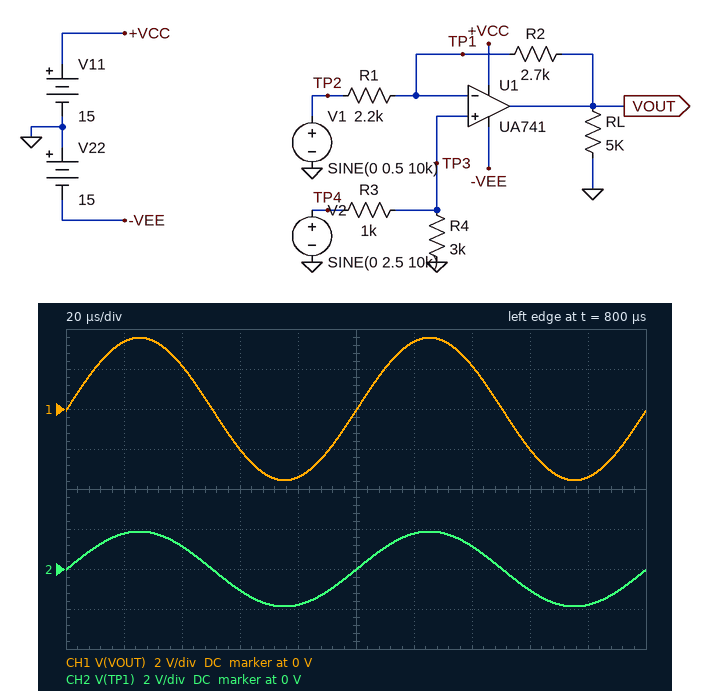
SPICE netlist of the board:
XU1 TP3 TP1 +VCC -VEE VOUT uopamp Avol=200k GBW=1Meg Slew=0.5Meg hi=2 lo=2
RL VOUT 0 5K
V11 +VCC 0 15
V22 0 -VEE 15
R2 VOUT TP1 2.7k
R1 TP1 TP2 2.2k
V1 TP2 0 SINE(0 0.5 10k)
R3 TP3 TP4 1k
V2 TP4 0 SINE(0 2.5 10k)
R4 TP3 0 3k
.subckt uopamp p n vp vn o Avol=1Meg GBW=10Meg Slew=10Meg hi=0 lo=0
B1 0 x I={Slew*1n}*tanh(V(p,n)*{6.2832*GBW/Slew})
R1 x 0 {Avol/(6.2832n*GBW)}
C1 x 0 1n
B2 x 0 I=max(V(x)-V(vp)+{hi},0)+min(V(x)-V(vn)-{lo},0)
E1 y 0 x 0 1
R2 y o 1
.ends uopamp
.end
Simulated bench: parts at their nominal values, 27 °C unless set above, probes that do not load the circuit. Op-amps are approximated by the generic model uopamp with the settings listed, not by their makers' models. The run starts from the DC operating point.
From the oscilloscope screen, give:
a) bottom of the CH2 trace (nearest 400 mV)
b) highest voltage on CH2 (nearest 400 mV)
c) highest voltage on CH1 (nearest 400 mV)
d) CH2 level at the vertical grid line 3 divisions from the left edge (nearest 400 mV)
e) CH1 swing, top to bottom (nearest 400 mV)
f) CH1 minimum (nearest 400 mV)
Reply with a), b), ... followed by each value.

a) -2.0 V
b) 2.0 V
c) 3.6 V
d) -1.2 V
e) 7.2 V
f) -3.6 V
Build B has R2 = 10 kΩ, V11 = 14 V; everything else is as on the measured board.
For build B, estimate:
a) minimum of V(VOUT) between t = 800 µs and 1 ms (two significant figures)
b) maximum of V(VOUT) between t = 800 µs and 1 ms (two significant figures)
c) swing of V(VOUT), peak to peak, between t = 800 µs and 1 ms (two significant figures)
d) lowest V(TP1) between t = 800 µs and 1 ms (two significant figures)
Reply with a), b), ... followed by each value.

a) -8.1 V
b) 8.1 V
c) 16 V
d) -1.9 V
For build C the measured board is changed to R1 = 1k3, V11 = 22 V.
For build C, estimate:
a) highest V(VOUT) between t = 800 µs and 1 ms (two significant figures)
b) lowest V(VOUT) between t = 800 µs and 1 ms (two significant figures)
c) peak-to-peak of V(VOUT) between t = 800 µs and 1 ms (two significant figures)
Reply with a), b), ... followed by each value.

a) 4.7 V
b) -4.7 V
c) 9.5 V
